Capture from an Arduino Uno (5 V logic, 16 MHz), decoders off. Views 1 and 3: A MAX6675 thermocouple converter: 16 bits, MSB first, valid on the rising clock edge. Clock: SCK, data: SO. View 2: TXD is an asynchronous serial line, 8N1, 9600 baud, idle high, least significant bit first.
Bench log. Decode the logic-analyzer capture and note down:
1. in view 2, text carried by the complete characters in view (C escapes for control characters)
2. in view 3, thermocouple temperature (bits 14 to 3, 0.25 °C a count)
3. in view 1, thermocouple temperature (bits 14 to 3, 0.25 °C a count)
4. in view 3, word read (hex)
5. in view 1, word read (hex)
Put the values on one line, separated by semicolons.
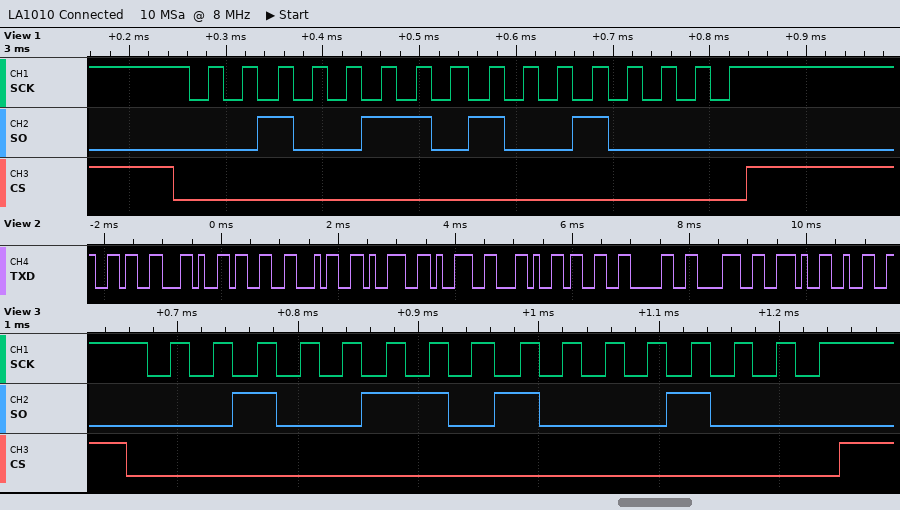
"6,3499,308.2"; 308.25 °C; 308.50 °C; 0x2688; 0x2690
